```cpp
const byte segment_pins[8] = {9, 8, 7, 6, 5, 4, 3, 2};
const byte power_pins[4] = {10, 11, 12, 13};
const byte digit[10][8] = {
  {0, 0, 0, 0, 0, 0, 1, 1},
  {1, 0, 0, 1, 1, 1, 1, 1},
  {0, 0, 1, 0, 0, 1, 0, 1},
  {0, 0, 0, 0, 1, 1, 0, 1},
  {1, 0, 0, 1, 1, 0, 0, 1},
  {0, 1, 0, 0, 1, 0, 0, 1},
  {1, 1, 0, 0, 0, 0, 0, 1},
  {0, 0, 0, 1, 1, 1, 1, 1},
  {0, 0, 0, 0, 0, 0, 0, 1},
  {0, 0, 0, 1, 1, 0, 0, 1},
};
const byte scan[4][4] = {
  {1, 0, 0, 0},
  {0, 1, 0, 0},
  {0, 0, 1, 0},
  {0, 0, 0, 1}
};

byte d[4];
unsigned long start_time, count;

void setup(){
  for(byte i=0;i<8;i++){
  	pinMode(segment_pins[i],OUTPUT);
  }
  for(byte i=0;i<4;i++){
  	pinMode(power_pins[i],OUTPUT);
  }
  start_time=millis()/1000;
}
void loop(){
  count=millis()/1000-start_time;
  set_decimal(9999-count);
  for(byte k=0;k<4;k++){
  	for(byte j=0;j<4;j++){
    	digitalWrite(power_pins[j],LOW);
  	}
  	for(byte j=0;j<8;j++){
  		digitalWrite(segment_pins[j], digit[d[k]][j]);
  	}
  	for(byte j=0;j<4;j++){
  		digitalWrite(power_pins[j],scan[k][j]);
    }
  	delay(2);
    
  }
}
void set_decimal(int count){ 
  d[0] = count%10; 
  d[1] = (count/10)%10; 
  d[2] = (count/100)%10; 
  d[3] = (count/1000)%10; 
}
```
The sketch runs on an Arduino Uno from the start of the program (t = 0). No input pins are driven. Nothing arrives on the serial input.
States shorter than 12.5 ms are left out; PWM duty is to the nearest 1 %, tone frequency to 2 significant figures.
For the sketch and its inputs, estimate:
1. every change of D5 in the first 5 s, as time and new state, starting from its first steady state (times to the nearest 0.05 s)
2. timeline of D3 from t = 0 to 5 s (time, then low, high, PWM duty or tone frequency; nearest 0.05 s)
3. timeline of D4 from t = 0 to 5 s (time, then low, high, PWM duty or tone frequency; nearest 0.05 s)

0 s high; 1 s tone 120 Hz; 2 s high; 3 s tone 120 Hz; 4 s high
0 s low; 2 s tone 120 Hz; 3 s low
0 s low; 2 s tone 120 Hz; 3 s low
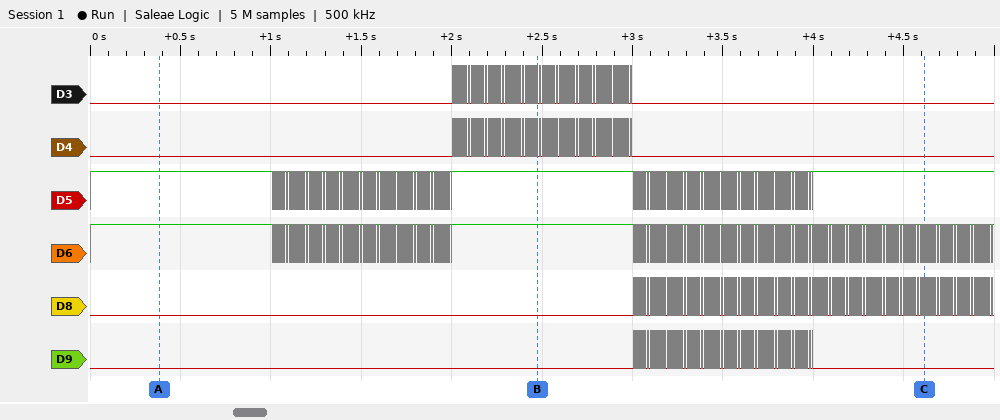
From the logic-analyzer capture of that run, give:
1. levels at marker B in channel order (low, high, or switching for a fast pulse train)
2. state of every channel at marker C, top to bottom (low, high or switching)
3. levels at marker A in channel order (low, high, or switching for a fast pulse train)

D3 switching, D4 switching, D5 high, D6 high, D8 low, D9 low
D3 low, D4 low, D5 high, D6 switching, D8 switching, D9 low
D3 low, D4 low, D5 high, D6 high, D8 low, D9 low
